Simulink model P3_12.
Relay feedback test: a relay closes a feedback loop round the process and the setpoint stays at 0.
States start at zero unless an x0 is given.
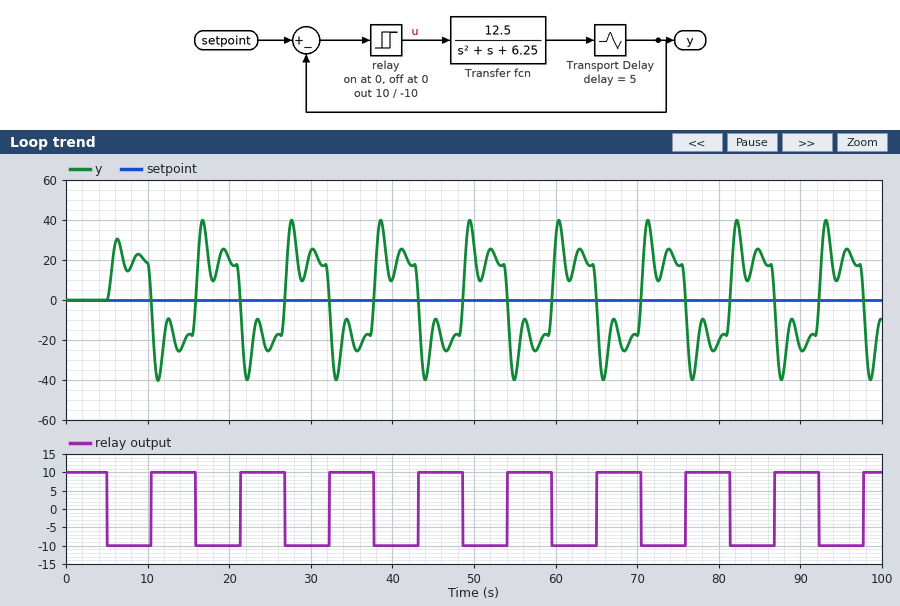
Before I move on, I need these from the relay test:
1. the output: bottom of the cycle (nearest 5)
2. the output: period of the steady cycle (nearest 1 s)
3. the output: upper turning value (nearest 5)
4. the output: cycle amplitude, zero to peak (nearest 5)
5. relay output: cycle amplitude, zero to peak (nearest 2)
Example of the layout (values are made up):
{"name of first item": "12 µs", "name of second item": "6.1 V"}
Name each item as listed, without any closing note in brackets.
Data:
{"the output: bottom of the cycle": "-40", "the output: period of the steady cycle": "11 s", "the output: upper turning value": "40", "the output: cycle amplitude, zero to peak": "40", "relay output: cycle amplitude, zero to peak": "10"}
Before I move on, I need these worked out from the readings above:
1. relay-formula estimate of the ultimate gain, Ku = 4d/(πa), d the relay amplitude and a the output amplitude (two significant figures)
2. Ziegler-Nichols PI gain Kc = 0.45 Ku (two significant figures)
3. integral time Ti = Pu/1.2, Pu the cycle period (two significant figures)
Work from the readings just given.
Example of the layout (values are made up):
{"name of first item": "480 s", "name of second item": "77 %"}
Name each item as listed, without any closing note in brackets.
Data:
{"relay-formula estimate of the ultimate gain, Ku = 4d/(πa), d the relay amplitude and a the output amplitude": "0.32", "Ziegler-Nichols PI gain Kc = 0.45 Ku": "0.14", "integral time Ti = Pu/1.2, Pu the cycle period": "9.2 s"}
